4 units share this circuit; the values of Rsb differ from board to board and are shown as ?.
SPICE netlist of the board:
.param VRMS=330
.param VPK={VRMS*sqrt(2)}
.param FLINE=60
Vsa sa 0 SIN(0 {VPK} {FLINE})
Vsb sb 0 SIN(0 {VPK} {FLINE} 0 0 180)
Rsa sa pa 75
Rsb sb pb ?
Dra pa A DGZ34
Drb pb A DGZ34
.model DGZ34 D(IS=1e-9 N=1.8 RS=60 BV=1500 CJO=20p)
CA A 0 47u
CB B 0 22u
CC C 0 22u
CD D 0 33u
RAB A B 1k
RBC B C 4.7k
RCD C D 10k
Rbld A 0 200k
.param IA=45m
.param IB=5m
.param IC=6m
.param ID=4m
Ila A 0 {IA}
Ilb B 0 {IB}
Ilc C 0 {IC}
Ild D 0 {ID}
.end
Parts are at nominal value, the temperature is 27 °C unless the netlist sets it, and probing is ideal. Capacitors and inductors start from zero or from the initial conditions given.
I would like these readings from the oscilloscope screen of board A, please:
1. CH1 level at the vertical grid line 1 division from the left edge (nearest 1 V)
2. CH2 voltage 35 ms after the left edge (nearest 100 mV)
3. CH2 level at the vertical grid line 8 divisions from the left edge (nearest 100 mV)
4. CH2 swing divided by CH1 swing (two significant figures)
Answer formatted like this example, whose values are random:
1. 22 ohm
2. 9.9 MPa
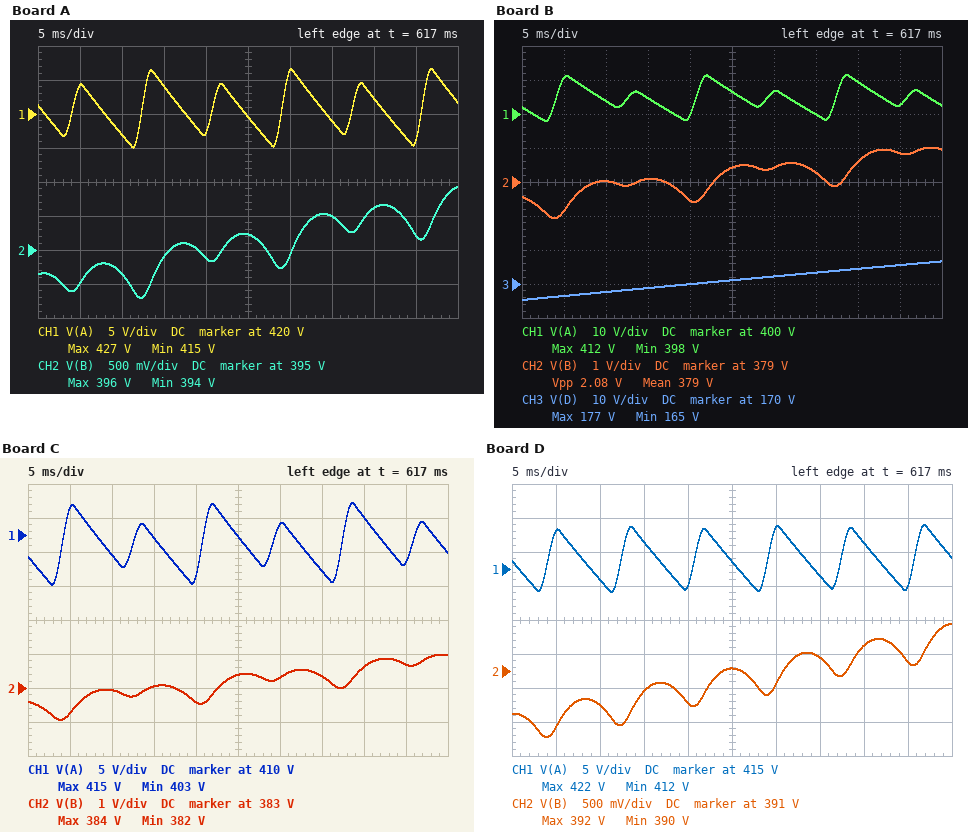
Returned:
1. 424 V
2. 395.5 V
3. 395.6 V
4. 0.14
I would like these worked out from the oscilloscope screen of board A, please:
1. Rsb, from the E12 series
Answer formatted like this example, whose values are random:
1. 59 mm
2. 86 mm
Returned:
1. 39 Ω
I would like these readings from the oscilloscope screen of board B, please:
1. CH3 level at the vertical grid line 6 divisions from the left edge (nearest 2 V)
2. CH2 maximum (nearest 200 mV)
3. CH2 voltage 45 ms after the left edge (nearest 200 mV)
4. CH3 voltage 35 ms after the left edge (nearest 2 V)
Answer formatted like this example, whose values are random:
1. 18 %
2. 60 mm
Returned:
1. 172 V
2. 380.0 V
3. 379.8 V
4. 174 V
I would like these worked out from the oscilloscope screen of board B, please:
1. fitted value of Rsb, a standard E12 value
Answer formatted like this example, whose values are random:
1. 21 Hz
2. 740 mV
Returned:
1. 220 Ω
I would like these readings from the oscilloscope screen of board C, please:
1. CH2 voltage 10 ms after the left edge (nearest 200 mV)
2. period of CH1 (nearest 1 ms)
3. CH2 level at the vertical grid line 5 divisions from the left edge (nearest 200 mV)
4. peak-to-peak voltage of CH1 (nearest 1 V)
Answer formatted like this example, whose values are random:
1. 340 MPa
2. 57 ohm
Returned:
1. 383.0 V
2. 8 ms
3. 383.4 V
4. 12 V
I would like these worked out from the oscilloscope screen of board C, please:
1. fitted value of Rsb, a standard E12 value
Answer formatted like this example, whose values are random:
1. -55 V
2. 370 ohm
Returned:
1. 150 Ω
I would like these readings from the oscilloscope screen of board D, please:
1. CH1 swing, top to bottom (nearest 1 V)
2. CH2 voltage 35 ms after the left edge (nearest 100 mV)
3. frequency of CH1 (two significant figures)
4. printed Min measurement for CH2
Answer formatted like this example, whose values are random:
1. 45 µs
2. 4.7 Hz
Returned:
1. 10 V
2. 391.2 V
3. 120 Hz
4. 390 V
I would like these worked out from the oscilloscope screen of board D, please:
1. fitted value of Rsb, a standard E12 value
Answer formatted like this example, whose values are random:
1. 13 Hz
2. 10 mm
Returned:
1. 68 Ω
